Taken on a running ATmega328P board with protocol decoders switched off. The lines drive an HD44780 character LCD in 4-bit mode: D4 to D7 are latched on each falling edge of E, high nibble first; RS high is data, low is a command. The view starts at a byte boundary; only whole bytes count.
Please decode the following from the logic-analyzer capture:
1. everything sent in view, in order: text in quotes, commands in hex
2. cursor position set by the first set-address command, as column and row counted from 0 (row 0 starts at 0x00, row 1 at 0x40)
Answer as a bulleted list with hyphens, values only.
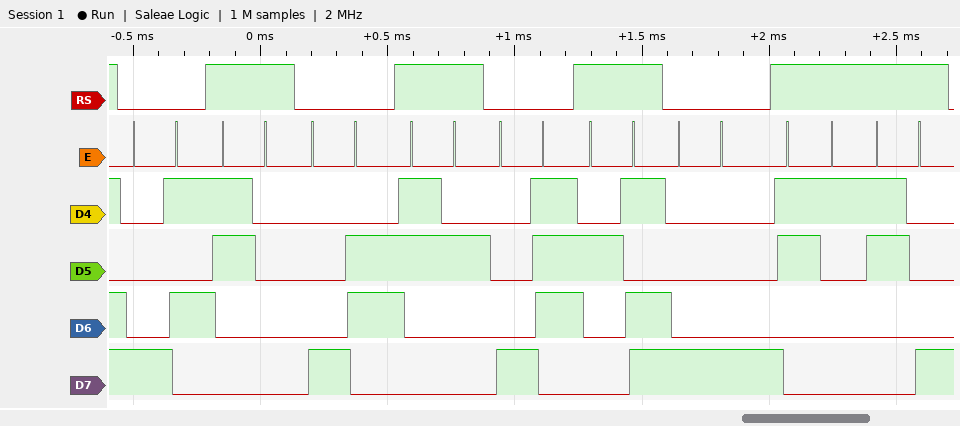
- 0x85 "0" 0x86 "2" 0x87 "-" 0x88 "18"
- column 5, row 0
